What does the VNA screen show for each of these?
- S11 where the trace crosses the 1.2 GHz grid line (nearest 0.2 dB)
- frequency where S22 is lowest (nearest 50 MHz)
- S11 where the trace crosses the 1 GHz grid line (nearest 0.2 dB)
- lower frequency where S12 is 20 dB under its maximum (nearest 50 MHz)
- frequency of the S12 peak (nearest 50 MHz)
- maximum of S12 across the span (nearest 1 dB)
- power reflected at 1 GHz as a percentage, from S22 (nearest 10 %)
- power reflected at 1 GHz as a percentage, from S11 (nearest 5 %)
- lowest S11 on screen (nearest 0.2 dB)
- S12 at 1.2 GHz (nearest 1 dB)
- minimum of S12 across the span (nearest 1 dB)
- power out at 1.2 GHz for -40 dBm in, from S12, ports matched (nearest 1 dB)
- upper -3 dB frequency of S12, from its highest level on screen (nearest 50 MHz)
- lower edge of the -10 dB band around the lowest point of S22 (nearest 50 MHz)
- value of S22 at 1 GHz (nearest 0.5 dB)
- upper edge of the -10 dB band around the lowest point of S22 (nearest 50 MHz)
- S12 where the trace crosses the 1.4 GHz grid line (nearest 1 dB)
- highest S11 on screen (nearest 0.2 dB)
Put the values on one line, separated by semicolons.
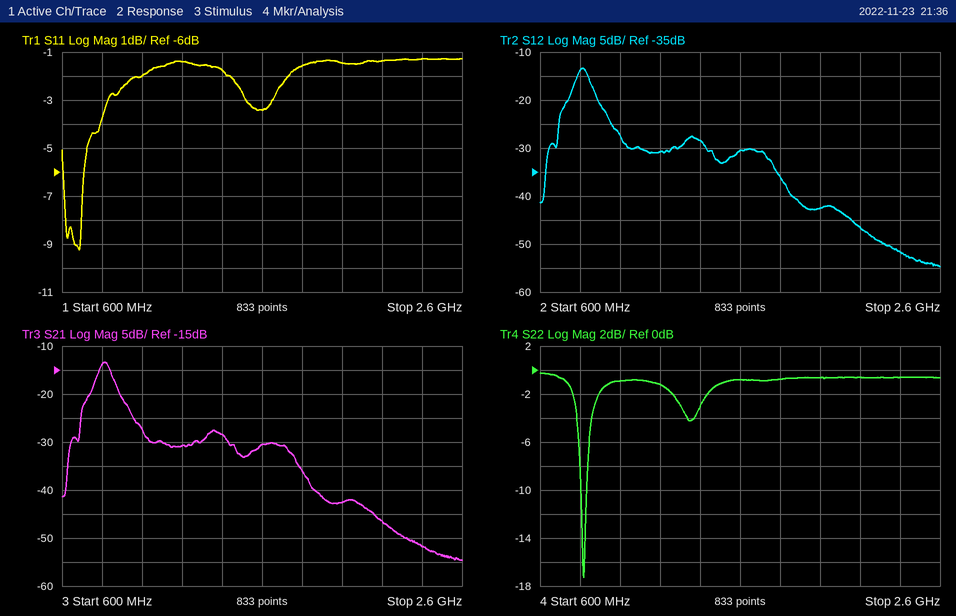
-1.4 dB; 800 MHz; -2.0 dB; 650 MHz; 800 MHz; -13 dB; 80 %; 65 %; -9.2 dB; -31 dB; -55 dB; -71 dBm; 850 MHz; 800 MHz; -1.0 dB; 850 MHz; -28 dB; -1.2 dB
